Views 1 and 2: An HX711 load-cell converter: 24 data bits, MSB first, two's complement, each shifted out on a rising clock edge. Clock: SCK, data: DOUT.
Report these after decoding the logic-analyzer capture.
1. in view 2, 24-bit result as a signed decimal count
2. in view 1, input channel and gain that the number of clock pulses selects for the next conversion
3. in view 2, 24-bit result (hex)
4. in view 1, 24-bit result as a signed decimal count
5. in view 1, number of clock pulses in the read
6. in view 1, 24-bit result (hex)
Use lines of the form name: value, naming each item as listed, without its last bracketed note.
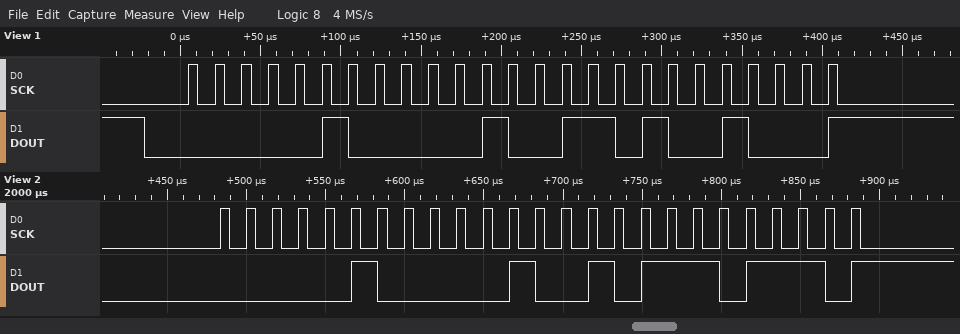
in view 2, 24-bit result as a signed decimal count: 266990
in view 1, input channel and gain that the number of clock pulses selects for the next conversion: channel A, gain 128
in view 2, 24-bit result: 0x0412EE
in view 1, 24-bit result as a signed decimal count: 267080
in view 1, number of clock pulses in the read: 25
in view 1, 24-bit result: 0x041348
